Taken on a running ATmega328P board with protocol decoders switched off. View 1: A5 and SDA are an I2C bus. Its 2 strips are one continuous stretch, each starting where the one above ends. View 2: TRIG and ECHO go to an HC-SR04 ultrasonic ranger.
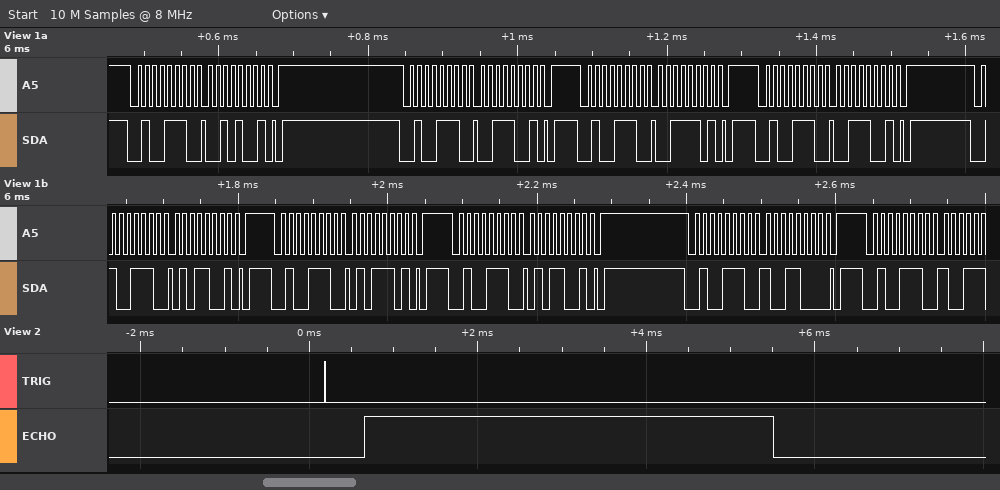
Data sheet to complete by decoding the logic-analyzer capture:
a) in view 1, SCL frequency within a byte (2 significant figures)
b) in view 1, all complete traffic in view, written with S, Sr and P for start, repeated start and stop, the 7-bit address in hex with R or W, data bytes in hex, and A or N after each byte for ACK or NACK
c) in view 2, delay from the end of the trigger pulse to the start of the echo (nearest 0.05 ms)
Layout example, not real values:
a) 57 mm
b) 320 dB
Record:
a) 100 kHz
b) S 27W A 29 A P S 27W A 39 A P S 27W A 3D A P S 27W A 39 A P S 27W A 59 A P S 27W A 5D A P S 27W A 59 A P S 27W A 98 A P S 27W A
c) 0.45 ms
